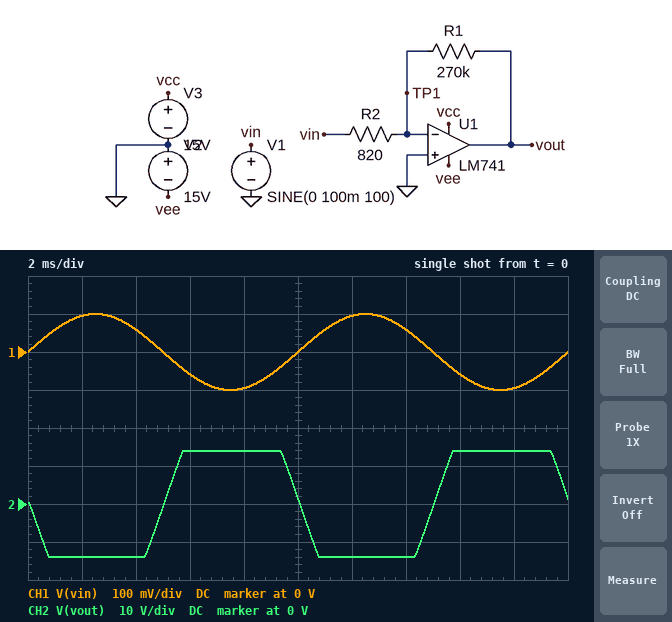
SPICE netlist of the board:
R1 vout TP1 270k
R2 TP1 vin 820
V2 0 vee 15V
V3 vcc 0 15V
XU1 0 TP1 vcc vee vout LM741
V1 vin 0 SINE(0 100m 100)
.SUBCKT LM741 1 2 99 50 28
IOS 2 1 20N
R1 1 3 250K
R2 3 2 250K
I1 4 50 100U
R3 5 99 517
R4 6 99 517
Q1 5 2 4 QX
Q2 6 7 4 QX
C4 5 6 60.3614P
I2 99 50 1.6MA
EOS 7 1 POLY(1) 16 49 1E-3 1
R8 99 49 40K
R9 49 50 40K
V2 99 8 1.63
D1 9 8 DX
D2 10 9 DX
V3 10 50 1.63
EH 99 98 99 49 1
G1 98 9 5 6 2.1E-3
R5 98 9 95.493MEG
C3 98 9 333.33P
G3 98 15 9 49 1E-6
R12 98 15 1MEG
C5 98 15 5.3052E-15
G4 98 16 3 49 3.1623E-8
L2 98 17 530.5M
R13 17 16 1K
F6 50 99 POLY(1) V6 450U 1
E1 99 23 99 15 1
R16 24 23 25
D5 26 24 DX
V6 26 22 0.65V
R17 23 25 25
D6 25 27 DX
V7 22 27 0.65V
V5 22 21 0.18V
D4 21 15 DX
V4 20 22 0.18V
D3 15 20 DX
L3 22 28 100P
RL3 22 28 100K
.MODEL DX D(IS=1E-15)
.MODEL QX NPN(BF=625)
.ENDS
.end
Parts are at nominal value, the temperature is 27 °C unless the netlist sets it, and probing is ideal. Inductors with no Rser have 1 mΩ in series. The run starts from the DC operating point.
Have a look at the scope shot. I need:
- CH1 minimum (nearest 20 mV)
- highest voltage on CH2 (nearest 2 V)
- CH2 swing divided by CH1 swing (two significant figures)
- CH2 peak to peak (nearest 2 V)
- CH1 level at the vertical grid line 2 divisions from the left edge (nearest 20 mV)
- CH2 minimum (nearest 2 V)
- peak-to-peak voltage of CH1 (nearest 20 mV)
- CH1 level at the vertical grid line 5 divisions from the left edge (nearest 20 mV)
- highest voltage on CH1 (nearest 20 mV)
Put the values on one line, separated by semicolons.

-100 mV; 14 V; 140; 28 V; 60 mV; -14 V; 200 mV; 0 V; 100 mV
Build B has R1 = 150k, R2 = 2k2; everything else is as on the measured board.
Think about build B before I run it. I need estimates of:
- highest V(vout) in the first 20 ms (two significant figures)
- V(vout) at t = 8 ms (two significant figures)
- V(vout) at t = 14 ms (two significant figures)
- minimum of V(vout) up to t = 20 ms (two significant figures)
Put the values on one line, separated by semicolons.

6.9 V; 6.6 V; -4.0 V; -6.7 V
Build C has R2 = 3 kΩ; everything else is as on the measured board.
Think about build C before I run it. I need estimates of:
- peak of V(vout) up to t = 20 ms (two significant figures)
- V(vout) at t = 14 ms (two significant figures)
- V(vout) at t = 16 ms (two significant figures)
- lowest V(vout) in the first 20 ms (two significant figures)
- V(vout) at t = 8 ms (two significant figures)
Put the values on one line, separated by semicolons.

9.1 V; -5.2 V; 5.3 V; -8.9 V; 8.7 V
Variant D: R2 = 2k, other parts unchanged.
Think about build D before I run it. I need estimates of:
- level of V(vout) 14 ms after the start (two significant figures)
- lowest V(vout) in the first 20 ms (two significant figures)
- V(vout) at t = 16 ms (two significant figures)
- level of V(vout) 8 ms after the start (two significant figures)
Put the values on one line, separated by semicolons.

-7.9 V; -13 V; 7.9 V; 13 V
